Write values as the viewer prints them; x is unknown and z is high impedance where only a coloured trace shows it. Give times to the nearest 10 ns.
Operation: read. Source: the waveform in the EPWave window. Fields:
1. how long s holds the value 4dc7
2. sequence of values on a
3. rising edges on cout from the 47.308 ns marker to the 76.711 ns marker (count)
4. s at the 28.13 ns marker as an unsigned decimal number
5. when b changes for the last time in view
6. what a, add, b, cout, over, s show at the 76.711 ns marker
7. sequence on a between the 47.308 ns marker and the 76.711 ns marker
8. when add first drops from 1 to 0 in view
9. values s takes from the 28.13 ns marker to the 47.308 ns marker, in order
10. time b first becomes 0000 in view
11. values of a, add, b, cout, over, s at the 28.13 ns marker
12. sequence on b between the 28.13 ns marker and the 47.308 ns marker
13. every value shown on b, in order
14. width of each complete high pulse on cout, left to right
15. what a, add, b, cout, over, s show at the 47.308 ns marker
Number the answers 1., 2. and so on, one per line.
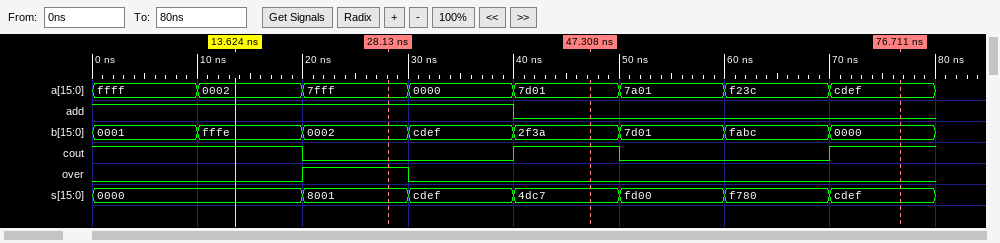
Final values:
1. 10 ns
2. ffff, 0002, 7fff, 0000, 7d01, 7a01, f23c, cdef
3. 1
4. 32769
5. 70 ns
6. a=cdef, add=0, b=0000, cout=1, over=0, s=cdef
7. 7d01, 7a01, f23c, cdef
8. 40 ns
9. 8001, cdef, 4dc7
10. 70 ns
11. a=7fff, add=1, b=0002, cout=0, over=1, s=8001
12. 0002, cdef, 2f3a
13. 0001, fffe, 0002, cdef, 2f3a, 7d01, fabc, 0000
14. 10 ns
15. a=7d01, add=0, b=2f3a, cout=1, over=0, s=4dc7
